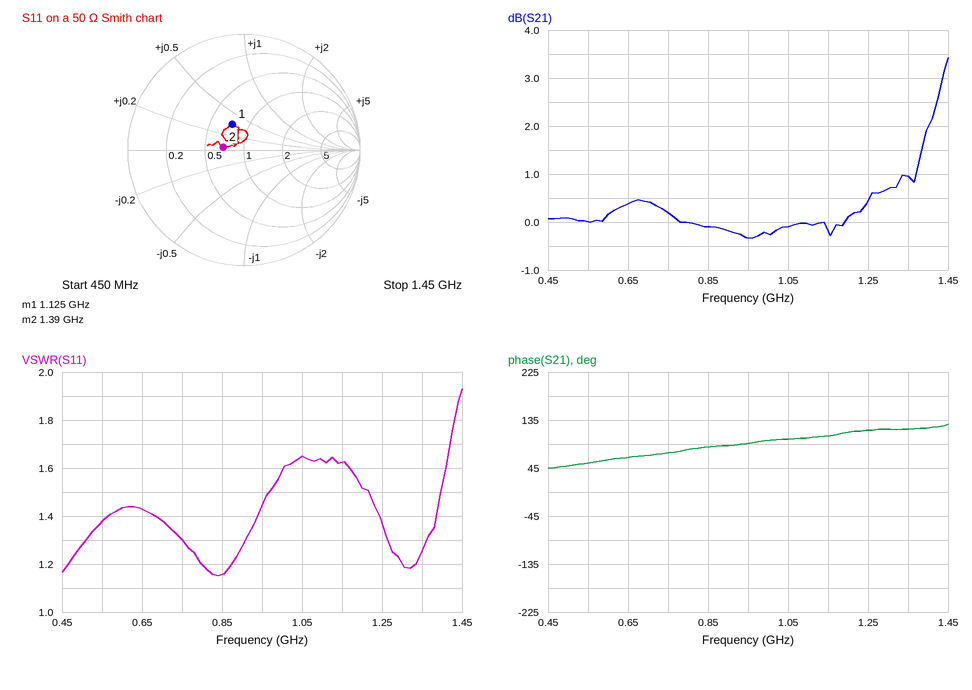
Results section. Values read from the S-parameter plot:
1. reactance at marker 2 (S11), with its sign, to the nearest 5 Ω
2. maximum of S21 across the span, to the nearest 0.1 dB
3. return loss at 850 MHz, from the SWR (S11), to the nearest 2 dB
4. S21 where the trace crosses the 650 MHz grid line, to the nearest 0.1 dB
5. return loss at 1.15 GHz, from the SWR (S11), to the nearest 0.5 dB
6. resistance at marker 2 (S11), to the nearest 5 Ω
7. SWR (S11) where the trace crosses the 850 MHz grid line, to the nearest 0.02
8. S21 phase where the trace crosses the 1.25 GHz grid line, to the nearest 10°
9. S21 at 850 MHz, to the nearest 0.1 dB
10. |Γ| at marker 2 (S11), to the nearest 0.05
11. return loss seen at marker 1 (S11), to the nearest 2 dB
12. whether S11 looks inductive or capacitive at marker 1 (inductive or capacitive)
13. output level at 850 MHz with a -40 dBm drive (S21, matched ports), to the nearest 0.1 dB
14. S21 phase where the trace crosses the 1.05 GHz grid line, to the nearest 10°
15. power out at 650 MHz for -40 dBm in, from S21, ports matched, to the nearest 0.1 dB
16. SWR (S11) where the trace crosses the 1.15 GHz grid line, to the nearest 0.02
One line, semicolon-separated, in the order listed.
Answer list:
0 Ω; 3.4 dB; 22 dB; 0.4 dB; 12.5 dB; 35 Ω; 1.16; 120°; -0.1 dB; 0.20; 12 dB; inductive; -40.1 dBm; 100°; -39.6 dBm; 1.62
